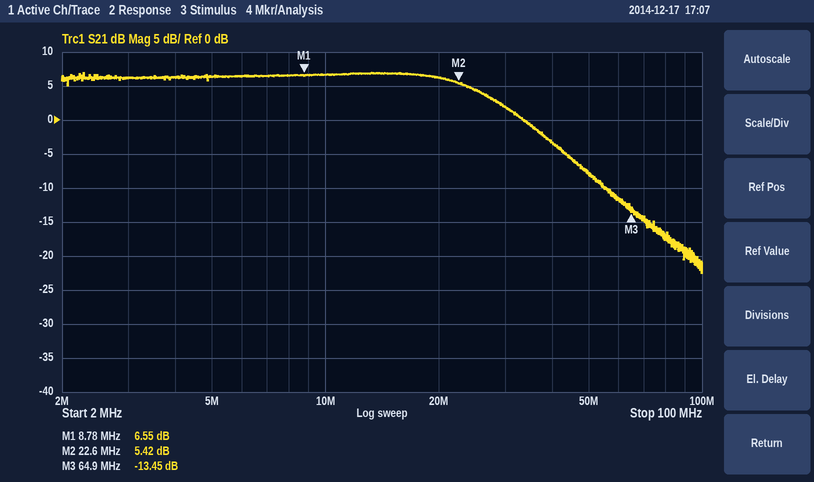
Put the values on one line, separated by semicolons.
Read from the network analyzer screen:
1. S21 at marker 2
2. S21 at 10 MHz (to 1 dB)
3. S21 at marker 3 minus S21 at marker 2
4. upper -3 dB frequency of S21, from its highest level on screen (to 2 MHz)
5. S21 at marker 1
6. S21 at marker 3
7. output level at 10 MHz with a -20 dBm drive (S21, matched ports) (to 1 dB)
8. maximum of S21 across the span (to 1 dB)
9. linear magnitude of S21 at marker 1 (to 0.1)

5.42 dB; 7 dB; -18.87 dB; 26 MHz; 6.55 dB; -13.45 dB; -13 dBm; 7 dB; 2.1
